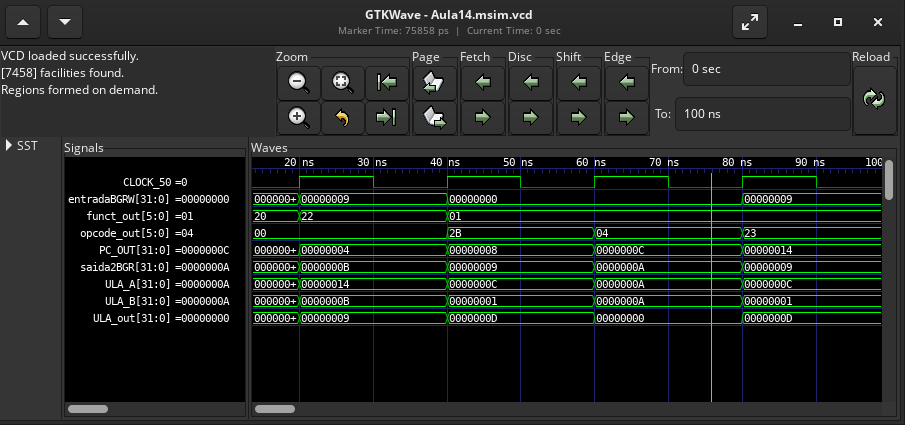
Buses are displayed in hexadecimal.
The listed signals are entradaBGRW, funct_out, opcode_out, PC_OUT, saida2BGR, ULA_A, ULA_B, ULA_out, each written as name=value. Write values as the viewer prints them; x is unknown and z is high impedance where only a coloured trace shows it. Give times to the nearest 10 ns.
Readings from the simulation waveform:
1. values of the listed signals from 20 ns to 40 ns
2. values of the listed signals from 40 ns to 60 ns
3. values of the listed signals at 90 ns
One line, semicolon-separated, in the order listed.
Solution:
entradaBGRW=00000009, funct_out=22, opcode_out=00, PC_OUT=00000004, saida2BGR=0000000B, ULA_A=00000014, ULA_B=0000000B, ULA_out=00000009; entradaBGRW=00000000, funct_out=01, opcode_out=2B, PC_OUT=00000008, saida2BGR=00000009, ULA_A=0000000C, ULA_B=00000001, ULA_out=0000000D; entradaBGRW=00000009, funct_out=01, opcode_out=23, PC_OUT=00000014, saida2BGR=00000009, ULA_A=0000000C, ULA_B=00000001, ULA_out=0000000D
